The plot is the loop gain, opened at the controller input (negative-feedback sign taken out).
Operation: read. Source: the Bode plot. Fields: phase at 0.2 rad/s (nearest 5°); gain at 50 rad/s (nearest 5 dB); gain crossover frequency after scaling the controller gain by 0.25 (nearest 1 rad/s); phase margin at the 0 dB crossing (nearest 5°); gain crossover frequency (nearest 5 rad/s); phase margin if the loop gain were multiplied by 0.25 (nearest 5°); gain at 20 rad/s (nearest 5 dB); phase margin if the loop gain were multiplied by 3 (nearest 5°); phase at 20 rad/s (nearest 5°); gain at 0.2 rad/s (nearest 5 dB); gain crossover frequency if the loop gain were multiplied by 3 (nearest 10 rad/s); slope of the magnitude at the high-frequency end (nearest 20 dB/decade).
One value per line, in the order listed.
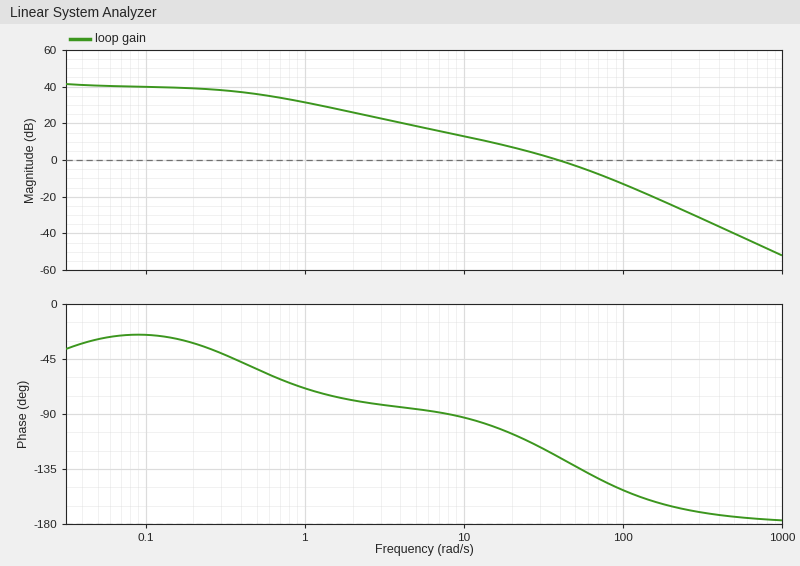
-30°
-5 dB
11 rad/s
55°
40 rad/s
85°
5 dB
35°
-105°
40 dB
80 rad/s
-40 dB/decade
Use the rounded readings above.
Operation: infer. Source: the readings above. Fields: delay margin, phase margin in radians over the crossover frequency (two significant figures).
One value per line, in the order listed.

0.024 s
